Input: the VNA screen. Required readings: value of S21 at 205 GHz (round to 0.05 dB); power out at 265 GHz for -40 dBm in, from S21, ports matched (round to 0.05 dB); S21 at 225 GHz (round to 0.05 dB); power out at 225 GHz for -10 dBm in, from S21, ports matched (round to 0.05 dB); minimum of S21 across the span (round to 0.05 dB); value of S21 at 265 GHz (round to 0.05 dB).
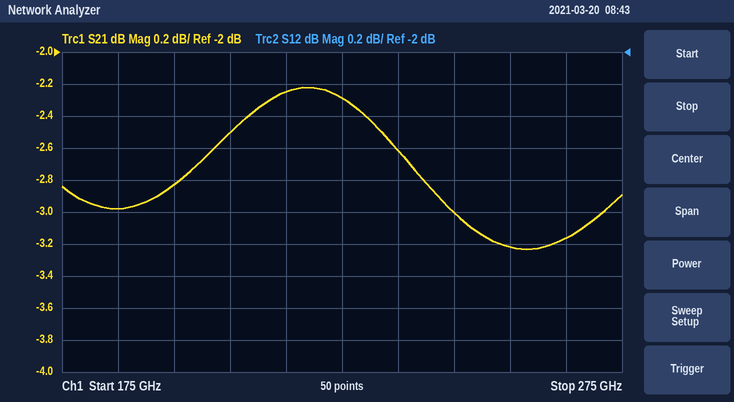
-2.50 dB
-43.15 dBm
-2.30 dB
-12.30 dBm
-3.25 dB
-3.15 dB
